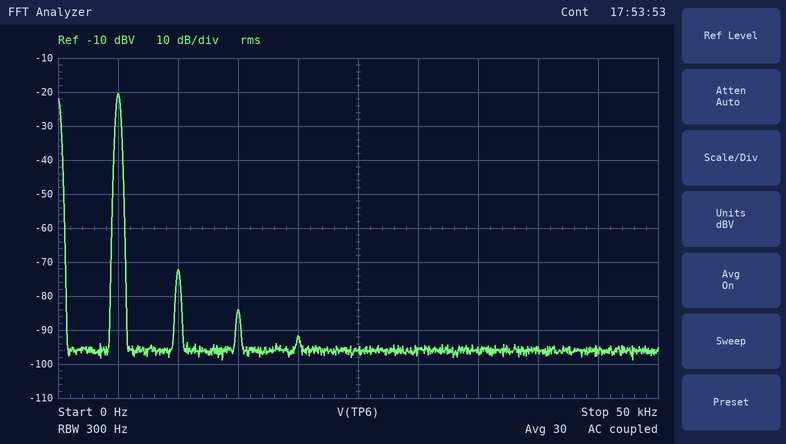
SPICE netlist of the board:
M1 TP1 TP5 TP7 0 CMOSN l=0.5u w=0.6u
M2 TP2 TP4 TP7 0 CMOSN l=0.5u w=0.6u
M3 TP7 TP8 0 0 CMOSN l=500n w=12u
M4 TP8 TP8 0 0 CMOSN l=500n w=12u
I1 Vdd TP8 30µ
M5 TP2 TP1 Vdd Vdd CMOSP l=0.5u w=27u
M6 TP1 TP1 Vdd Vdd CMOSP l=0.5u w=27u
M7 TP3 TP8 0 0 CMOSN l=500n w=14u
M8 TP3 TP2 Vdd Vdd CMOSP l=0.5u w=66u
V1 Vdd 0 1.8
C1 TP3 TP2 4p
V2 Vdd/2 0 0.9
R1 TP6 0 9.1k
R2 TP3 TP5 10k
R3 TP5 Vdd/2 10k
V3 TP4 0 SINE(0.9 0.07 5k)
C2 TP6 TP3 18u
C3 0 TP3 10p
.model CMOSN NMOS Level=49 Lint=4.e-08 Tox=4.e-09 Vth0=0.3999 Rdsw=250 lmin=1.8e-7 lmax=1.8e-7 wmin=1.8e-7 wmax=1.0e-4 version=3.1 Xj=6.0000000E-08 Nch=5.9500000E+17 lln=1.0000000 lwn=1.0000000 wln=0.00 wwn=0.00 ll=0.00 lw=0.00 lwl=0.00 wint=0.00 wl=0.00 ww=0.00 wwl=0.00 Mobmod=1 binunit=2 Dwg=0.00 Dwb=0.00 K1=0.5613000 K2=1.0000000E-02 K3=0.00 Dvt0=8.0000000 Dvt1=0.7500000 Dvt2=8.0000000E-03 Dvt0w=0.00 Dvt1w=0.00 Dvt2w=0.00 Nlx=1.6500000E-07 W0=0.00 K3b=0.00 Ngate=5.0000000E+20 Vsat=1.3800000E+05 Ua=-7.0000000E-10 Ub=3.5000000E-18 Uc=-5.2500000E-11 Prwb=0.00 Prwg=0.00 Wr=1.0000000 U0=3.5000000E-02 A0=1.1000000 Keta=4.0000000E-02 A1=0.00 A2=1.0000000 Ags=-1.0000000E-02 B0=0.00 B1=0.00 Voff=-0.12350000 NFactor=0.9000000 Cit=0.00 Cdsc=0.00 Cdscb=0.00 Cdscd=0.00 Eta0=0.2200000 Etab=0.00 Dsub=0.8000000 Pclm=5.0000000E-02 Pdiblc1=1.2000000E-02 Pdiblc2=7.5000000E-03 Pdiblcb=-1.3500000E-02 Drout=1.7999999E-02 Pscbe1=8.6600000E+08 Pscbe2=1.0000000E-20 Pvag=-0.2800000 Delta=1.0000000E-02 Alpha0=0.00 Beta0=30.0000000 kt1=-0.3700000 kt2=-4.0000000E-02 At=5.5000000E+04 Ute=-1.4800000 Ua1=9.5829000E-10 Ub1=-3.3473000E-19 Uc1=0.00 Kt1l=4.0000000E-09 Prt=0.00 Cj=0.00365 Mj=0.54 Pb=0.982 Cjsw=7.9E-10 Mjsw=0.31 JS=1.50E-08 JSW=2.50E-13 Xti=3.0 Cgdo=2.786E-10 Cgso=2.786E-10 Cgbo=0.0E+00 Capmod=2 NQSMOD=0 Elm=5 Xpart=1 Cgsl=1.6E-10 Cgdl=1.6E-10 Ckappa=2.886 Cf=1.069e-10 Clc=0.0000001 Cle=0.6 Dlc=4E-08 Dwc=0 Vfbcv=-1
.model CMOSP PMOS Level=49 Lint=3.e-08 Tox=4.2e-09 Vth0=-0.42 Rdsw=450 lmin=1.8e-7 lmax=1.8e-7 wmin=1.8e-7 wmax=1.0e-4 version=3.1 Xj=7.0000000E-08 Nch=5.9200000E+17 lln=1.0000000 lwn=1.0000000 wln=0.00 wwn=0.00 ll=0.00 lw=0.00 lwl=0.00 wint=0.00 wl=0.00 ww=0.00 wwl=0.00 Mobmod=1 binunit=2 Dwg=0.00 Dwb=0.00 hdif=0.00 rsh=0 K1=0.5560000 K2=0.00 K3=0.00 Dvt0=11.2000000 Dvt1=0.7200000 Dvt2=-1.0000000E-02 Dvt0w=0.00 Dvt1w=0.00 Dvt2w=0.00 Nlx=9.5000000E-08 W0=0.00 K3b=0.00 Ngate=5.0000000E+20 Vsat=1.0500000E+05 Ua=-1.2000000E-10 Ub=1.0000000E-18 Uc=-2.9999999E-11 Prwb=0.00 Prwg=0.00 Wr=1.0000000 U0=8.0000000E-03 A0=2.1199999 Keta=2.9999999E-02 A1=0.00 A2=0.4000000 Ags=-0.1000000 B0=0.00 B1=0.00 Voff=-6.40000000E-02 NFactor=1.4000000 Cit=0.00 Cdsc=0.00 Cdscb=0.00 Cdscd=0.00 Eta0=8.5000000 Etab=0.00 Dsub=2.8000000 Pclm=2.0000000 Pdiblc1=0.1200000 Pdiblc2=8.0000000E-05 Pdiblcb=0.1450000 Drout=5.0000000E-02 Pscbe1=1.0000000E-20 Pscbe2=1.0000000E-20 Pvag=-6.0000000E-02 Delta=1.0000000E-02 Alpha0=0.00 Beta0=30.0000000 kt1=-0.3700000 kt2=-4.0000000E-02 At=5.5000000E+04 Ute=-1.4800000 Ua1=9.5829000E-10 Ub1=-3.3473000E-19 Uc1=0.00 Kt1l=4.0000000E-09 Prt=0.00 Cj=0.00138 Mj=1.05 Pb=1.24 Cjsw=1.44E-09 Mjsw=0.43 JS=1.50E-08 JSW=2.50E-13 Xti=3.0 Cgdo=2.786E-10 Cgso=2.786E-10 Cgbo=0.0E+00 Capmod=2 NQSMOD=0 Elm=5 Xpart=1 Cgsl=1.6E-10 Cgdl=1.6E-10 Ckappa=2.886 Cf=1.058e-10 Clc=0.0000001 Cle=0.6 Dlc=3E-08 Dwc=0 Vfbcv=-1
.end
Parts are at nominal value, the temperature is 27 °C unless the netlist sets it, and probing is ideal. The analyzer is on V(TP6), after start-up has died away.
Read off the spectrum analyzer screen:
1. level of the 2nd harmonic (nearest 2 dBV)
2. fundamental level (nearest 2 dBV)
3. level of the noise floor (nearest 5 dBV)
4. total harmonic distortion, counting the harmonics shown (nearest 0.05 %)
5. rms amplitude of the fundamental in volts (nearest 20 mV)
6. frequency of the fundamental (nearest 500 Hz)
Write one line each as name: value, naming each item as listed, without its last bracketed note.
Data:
level of the 2nd harmonic: -72 dBV
fundamental level: -20 dBV
level of the noise floor: -95 dBV
total harmonic distortion, counting the harmonics shown: 0.25 %
rms amplitude of the fundamental in volts: 100 mV
frequency of the fundamental: 5.0 kHz
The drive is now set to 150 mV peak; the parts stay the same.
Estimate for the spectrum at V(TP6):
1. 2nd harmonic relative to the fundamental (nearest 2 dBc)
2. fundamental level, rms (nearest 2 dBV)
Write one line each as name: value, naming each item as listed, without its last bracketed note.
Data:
2nd harmonic relative to the fundamental: -24 dBc
fundamental level, rms: -14 dBV
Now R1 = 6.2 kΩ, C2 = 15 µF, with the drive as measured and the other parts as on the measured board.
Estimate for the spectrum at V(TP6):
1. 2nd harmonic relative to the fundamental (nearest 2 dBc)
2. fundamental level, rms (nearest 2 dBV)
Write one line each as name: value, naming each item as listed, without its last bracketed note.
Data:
2nd harmonic relative to the fundamental: -44 dBc
fundamental level, rms: -20 dBV
